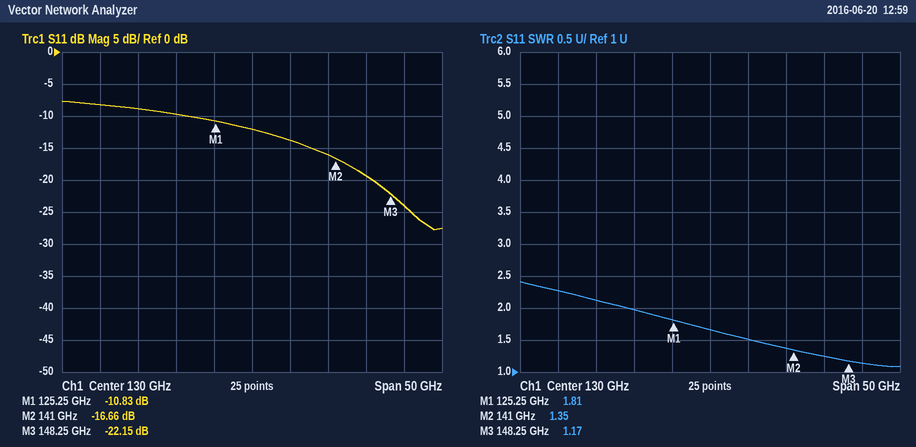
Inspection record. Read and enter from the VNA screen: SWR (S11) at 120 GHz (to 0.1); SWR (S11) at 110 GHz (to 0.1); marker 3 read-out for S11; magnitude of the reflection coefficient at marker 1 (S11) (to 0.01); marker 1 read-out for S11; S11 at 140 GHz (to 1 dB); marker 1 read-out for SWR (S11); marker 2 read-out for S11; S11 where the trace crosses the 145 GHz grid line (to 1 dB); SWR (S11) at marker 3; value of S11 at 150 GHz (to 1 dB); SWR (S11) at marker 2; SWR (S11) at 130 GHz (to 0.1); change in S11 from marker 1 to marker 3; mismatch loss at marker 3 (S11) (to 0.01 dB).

2.0
2.3
-22.15 dB
0.29
-10.83 dB
-16 dB
1.81
-16.66 dB
-19 dB
1.17
-24 dB
1.35
1.7
-11.32 dB
0.03 dB
